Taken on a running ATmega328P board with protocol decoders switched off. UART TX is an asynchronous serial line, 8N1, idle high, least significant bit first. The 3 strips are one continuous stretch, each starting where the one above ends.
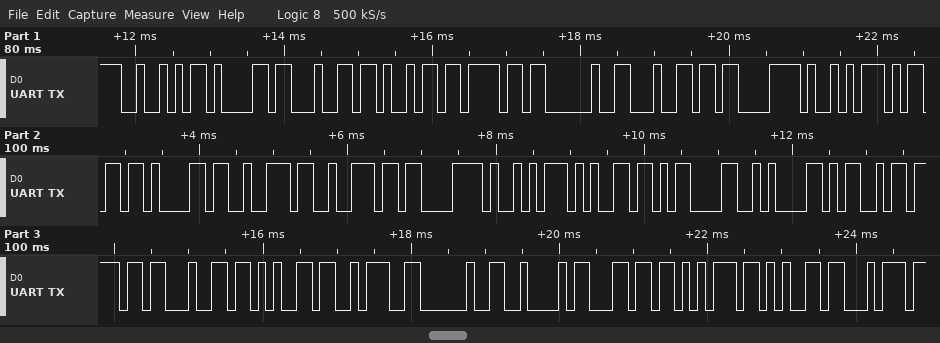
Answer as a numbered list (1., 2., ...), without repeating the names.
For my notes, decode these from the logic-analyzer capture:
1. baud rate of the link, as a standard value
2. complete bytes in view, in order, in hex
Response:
1. 9600 baud
2. 52 61 64 69 6F 20 64 C3 A9 6D 61 72 72 C3 A9 65 0D 0A 4D 6F 64 65 3A 20 42 6C 75 65 74
